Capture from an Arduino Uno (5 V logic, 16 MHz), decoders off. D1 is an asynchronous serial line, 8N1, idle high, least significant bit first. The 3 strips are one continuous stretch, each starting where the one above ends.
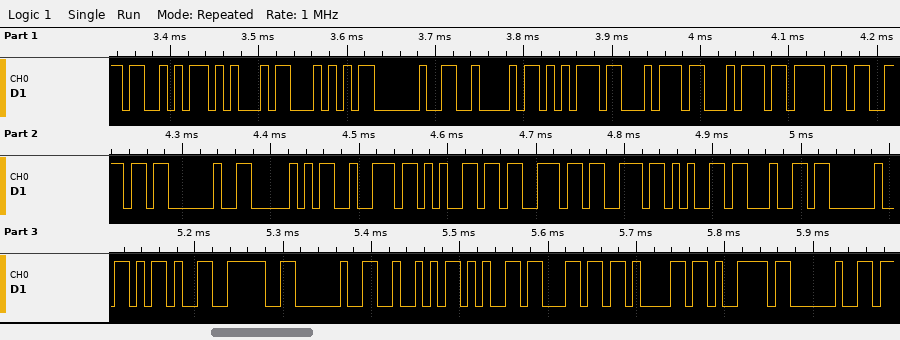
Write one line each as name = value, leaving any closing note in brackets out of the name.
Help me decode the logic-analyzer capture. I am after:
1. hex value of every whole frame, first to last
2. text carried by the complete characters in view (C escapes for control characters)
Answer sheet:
hex value of every whole frame, first to last = 0x53 0x45 0x54 0x20 0x42 0x75 0x74 0x74 0x6F 0x6E 0x20 0x50 0x72 0x65 0x73 0x73 0x65 0x64 0x20 0x2D 0x3E 0x20 0x52 0x65 0x6C 0x61 0x79 0x20
text carried by the complete characters in view = "SET Button Pressed -> Relay "
